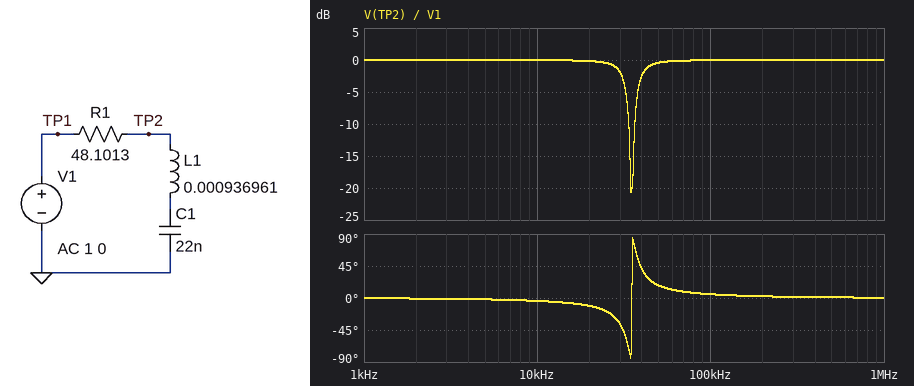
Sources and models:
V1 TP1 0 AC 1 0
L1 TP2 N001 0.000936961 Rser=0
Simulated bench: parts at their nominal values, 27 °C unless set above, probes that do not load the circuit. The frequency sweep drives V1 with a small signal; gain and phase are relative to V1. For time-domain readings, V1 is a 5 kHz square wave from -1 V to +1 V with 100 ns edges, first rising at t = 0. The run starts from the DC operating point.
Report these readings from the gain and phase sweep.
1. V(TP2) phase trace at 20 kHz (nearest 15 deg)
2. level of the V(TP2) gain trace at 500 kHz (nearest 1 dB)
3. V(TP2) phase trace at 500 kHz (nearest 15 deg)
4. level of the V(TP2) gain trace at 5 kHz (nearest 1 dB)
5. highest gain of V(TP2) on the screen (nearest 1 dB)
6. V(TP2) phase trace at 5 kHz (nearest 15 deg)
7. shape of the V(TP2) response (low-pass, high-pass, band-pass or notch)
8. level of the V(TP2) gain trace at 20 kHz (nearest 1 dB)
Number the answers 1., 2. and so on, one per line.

1. -15 deg
2. 0 dB
3. 0 deg
4. 0 dB
5. 0 dB
6. 0 deg
7. notch
8. 0 dB
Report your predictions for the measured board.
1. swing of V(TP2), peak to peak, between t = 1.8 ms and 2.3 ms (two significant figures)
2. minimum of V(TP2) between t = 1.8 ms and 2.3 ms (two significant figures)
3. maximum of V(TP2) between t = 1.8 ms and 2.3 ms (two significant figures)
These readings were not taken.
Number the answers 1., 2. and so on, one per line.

1. 2.6 V
2. -1.3 V
3. 1.3 V
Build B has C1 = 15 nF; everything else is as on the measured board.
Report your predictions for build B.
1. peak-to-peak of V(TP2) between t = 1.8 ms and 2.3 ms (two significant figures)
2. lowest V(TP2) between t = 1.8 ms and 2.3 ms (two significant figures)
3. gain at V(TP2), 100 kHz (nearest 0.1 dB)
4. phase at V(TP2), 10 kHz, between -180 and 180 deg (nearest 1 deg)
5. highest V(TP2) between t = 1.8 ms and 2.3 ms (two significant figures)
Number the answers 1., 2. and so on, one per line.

1. 2.5 V
2. -1.2 V
3. 0 dB
4. -3 deg
5. 1.2 V
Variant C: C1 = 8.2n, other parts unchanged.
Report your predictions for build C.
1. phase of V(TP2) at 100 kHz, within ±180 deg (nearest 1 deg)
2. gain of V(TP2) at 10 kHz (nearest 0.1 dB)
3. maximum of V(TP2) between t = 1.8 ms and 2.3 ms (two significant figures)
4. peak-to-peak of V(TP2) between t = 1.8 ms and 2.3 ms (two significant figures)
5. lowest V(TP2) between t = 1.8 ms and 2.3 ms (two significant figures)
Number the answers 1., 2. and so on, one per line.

1. 7 deg
2. 0 dB
3. 1.2 V
4. 2.4 V
5. -1.2 V
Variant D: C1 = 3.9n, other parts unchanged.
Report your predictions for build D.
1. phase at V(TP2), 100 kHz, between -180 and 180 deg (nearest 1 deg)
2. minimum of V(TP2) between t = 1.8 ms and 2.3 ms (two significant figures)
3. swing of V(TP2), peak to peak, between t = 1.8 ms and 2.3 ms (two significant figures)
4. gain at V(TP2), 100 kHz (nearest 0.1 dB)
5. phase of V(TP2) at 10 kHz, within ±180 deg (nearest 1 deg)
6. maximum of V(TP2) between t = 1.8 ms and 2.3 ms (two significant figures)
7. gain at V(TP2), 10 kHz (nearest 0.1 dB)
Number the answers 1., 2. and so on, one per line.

1. 15 deg
2. -1.2 V
3. 2.3 V
4. -0.3 dB
5. -1 deg
6. 1.2 V
7. 0 dB
